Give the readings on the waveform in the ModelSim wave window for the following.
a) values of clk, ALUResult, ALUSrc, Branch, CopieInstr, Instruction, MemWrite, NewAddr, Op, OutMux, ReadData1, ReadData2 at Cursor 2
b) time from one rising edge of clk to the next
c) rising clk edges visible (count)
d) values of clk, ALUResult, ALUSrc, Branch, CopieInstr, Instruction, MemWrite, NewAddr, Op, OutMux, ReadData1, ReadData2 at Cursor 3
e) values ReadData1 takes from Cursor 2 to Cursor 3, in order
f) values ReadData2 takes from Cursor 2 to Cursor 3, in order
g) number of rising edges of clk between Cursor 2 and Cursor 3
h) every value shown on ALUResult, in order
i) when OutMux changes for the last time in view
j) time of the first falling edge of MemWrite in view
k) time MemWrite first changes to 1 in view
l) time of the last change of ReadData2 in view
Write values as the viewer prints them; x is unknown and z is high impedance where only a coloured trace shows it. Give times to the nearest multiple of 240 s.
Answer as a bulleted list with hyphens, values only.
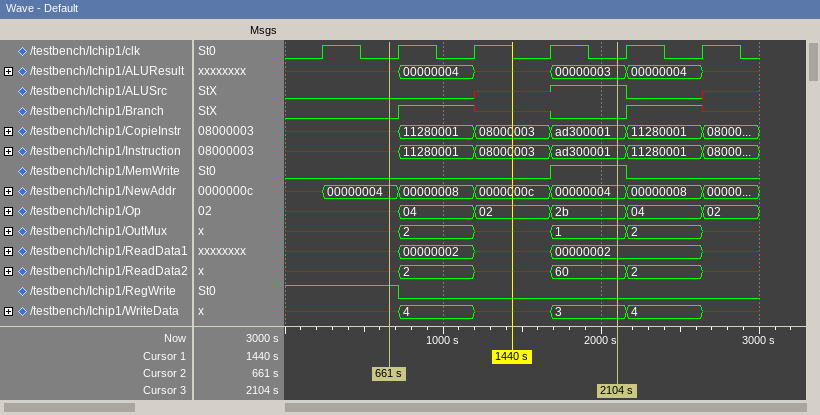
- clk=0, ALUResult=x, ALUSrc=0, Branch=0, CopieInstr=x, Instruction=x, MemWrite=0, NewAddr=00000004, Op=x, OutMux=x, ReadData1=x, ReadData2=x
- 480 s
- 6
- clk=0, ALUResult=00000003, ALUSrc=1, Branch=0, CopieInstr=ad300001, Instruction=ad300001, MemWrite=1, NewAddr=00000004, Op=2b, OutMux=1, ReadData1=00000002, ReadData2=60
- x, 00000002, x, 00000002
- x, 2, x, 60
- 3
- x, 00000004, x, 00000003, 00000004, x
- 2640 s
- 2160 s
- 1680 s
- 2640 s
